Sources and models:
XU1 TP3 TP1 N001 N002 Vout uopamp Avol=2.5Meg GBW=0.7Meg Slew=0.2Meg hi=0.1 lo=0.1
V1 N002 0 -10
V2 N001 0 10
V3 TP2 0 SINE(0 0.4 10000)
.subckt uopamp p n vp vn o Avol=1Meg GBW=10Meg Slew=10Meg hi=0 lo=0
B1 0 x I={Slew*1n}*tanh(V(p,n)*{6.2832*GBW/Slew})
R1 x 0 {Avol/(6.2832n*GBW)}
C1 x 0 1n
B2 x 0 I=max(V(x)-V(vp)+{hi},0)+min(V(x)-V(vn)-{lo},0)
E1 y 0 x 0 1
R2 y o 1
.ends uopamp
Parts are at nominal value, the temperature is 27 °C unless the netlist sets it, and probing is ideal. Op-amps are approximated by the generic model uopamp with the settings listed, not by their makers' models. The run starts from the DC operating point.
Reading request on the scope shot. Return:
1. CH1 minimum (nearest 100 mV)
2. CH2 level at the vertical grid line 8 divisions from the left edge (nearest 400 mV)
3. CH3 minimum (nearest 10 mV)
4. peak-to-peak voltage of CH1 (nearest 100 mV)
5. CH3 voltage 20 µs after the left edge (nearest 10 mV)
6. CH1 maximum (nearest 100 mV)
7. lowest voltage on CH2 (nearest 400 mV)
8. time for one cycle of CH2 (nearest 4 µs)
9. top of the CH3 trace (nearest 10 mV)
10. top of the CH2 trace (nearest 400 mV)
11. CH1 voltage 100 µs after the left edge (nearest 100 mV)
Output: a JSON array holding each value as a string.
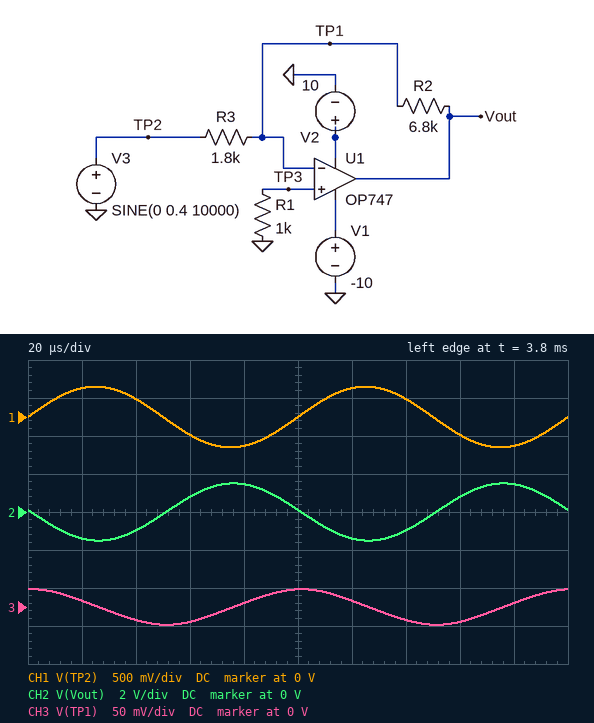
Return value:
["-400 mV", "800 mV", "-20 mV", "800 mV", "10 mV", "400 mV", "-1.6 V", "100 µs", "20 mV", "1.6 V", "0 V"]
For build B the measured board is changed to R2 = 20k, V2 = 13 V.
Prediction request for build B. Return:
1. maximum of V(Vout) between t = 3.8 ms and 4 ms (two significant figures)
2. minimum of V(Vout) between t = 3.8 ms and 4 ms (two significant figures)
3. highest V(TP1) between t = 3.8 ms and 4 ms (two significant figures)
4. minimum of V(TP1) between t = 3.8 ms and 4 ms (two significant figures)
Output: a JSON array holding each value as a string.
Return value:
["4.2 V", "-4.2 V", "170 mV", "-170 mV"]
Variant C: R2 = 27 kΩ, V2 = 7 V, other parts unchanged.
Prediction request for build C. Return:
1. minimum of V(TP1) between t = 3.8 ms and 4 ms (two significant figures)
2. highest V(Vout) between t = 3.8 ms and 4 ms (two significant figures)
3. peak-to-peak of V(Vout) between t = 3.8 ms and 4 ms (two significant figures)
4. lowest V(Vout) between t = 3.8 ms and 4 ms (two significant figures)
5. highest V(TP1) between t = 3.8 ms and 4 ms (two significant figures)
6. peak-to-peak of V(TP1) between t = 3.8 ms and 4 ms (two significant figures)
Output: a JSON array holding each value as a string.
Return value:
["-260 mV", "4.6 V", "9.1 V", "-4.6 V", "260 mV", "530 mV"]
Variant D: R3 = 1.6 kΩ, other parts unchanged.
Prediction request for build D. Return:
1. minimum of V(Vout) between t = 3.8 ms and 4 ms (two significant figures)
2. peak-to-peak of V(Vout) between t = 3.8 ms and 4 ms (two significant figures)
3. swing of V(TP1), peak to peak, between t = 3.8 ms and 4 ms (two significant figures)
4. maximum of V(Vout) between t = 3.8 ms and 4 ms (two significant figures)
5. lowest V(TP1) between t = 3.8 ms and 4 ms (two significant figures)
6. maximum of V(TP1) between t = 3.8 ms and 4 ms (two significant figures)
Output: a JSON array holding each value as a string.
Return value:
["-1.7 V", "3.4 V", "54 mV", "1.7 V", "-27 mV", "27 mV"]
